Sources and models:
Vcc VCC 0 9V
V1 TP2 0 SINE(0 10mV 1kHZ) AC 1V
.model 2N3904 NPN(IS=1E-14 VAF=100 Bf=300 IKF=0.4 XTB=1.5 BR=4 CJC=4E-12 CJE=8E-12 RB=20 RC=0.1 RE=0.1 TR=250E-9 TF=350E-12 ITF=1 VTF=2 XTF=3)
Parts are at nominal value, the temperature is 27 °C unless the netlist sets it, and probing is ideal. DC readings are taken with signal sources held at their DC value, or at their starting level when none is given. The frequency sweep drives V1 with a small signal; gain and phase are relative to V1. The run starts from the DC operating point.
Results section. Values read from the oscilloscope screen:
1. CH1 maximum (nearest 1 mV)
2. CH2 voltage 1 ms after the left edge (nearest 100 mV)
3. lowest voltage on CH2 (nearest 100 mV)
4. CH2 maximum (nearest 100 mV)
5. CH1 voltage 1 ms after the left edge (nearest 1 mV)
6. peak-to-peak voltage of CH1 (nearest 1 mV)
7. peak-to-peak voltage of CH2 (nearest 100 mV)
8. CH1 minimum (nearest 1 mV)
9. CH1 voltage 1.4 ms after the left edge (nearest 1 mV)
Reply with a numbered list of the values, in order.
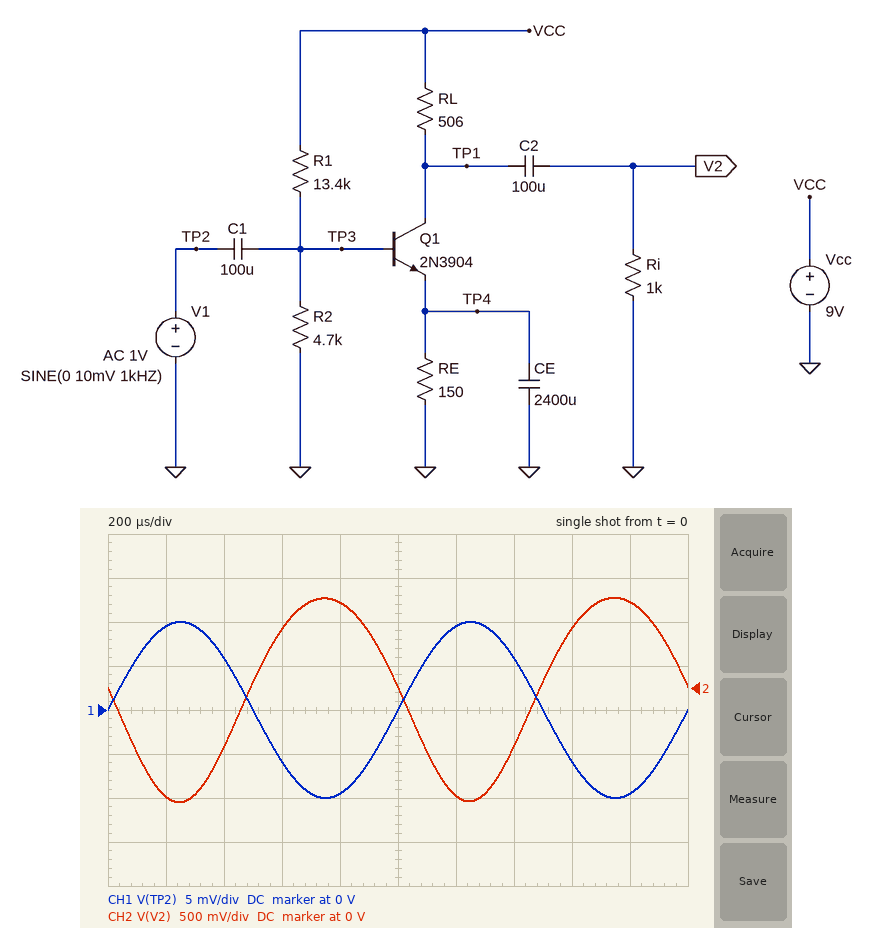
1. 10 mV
2. 0 V
3. -1.3 V
4. 1.0 V
5. 0 V
6. 20 mV
7. 2.3 V
8. -10 mV
9. 6 mV
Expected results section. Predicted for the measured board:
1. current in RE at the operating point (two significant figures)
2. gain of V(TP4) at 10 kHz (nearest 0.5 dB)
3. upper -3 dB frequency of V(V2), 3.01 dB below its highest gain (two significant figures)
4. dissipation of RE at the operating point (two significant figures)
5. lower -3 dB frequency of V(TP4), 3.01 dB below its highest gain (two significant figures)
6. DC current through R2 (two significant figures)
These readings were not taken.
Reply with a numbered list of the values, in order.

1. 10 mA
2. -53.0 dB
3. 17 MHz
4. 15 mW
5. 440 mHz
6. 470 µA
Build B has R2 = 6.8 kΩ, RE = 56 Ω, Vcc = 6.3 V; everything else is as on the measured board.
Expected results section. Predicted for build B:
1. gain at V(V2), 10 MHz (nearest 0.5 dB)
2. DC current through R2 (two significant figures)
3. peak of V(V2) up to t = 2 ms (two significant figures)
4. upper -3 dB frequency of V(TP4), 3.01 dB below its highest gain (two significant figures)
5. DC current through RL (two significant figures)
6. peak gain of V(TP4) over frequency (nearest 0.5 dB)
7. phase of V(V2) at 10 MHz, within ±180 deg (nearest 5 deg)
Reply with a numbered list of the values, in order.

1. -15.5 dB
2. 200 µA
3. 740 mV
4. 56 Hz
5. 11 mA
6. -24.5 dB
7. 50 deg
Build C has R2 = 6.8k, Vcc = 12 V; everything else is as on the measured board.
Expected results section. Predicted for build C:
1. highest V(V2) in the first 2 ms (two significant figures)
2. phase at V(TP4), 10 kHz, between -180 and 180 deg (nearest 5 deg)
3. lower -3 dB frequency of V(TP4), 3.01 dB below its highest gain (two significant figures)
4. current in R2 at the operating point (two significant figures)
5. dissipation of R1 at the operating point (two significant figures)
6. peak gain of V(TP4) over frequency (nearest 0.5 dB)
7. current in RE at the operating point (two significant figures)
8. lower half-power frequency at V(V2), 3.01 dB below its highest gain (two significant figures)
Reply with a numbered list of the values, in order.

1. 1.5 V
2. -90 deg
3. 800 mHz
4. 510 µA
5. 5.4 mW
6. -22.0 dB
7. 18 mA
8. 60 Hz
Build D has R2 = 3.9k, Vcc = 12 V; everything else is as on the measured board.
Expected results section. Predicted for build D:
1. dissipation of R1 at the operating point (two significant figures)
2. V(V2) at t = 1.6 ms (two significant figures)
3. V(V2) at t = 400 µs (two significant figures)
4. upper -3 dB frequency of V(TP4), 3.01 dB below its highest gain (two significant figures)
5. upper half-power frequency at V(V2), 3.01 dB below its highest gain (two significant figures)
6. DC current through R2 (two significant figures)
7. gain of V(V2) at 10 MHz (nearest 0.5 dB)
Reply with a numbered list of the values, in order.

1. 6.6 mW
2. 830 mV
3. -790 mV
4. 31 Hz
5. 16 MHz
6. 660 µA
7. 41.5 dB
